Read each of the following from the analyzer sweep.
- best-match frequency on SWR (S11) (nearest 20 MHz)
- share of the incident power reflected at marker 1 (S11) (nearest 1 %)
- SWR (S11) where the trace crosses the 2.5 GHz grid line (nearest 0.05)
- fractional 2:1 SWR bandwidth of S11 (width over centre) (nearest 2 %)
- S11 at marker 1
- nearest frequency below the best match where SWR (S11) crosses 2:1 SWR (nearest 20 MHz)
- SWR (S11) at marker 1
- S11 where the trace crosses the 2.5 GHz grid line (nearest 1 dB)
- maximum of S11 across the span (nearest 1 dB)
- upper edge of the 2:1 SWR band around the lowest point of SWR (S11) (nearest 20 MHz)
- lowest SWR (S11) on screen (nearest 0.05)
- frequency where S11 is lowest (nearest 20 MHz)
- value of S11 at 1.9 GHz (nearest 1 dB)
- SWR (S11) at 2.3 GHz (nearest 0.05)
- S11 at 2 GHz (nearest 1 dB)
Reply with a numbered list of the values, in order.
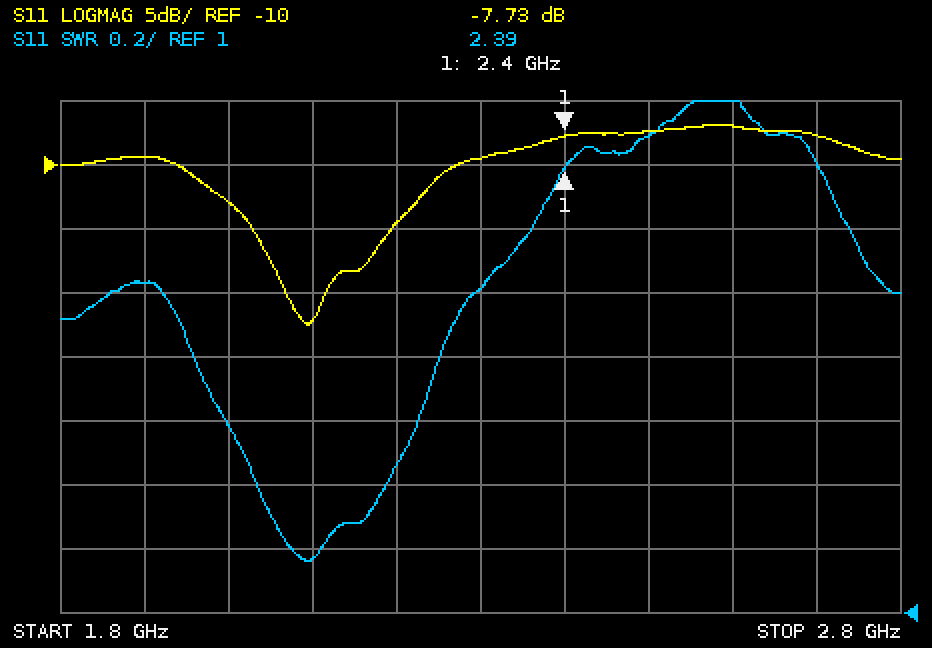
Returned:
1. 2.10 GHz
2. 17 %
3. 2.50
4. 18 %
5. -7.73 dB
6. 1.92 GHz
7. 2.39
8. -7 dB
9. -7 dB
10. 2.30 GHz
11. 1.15
12. 2.10 GHz
13. -9 dB
14. 2.00
15. -13 dB
